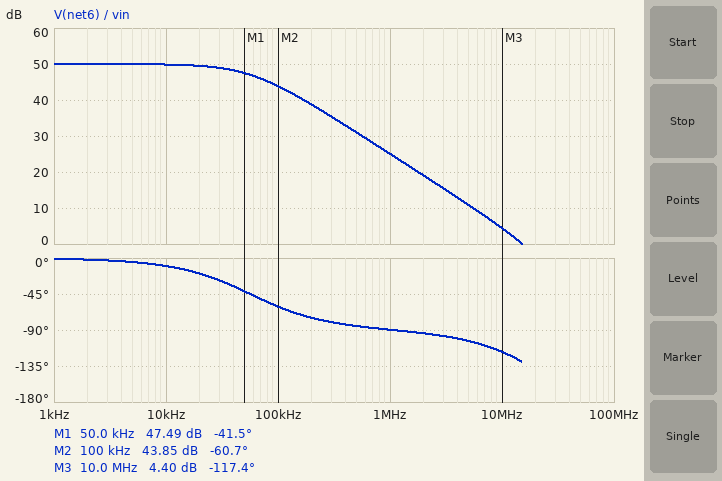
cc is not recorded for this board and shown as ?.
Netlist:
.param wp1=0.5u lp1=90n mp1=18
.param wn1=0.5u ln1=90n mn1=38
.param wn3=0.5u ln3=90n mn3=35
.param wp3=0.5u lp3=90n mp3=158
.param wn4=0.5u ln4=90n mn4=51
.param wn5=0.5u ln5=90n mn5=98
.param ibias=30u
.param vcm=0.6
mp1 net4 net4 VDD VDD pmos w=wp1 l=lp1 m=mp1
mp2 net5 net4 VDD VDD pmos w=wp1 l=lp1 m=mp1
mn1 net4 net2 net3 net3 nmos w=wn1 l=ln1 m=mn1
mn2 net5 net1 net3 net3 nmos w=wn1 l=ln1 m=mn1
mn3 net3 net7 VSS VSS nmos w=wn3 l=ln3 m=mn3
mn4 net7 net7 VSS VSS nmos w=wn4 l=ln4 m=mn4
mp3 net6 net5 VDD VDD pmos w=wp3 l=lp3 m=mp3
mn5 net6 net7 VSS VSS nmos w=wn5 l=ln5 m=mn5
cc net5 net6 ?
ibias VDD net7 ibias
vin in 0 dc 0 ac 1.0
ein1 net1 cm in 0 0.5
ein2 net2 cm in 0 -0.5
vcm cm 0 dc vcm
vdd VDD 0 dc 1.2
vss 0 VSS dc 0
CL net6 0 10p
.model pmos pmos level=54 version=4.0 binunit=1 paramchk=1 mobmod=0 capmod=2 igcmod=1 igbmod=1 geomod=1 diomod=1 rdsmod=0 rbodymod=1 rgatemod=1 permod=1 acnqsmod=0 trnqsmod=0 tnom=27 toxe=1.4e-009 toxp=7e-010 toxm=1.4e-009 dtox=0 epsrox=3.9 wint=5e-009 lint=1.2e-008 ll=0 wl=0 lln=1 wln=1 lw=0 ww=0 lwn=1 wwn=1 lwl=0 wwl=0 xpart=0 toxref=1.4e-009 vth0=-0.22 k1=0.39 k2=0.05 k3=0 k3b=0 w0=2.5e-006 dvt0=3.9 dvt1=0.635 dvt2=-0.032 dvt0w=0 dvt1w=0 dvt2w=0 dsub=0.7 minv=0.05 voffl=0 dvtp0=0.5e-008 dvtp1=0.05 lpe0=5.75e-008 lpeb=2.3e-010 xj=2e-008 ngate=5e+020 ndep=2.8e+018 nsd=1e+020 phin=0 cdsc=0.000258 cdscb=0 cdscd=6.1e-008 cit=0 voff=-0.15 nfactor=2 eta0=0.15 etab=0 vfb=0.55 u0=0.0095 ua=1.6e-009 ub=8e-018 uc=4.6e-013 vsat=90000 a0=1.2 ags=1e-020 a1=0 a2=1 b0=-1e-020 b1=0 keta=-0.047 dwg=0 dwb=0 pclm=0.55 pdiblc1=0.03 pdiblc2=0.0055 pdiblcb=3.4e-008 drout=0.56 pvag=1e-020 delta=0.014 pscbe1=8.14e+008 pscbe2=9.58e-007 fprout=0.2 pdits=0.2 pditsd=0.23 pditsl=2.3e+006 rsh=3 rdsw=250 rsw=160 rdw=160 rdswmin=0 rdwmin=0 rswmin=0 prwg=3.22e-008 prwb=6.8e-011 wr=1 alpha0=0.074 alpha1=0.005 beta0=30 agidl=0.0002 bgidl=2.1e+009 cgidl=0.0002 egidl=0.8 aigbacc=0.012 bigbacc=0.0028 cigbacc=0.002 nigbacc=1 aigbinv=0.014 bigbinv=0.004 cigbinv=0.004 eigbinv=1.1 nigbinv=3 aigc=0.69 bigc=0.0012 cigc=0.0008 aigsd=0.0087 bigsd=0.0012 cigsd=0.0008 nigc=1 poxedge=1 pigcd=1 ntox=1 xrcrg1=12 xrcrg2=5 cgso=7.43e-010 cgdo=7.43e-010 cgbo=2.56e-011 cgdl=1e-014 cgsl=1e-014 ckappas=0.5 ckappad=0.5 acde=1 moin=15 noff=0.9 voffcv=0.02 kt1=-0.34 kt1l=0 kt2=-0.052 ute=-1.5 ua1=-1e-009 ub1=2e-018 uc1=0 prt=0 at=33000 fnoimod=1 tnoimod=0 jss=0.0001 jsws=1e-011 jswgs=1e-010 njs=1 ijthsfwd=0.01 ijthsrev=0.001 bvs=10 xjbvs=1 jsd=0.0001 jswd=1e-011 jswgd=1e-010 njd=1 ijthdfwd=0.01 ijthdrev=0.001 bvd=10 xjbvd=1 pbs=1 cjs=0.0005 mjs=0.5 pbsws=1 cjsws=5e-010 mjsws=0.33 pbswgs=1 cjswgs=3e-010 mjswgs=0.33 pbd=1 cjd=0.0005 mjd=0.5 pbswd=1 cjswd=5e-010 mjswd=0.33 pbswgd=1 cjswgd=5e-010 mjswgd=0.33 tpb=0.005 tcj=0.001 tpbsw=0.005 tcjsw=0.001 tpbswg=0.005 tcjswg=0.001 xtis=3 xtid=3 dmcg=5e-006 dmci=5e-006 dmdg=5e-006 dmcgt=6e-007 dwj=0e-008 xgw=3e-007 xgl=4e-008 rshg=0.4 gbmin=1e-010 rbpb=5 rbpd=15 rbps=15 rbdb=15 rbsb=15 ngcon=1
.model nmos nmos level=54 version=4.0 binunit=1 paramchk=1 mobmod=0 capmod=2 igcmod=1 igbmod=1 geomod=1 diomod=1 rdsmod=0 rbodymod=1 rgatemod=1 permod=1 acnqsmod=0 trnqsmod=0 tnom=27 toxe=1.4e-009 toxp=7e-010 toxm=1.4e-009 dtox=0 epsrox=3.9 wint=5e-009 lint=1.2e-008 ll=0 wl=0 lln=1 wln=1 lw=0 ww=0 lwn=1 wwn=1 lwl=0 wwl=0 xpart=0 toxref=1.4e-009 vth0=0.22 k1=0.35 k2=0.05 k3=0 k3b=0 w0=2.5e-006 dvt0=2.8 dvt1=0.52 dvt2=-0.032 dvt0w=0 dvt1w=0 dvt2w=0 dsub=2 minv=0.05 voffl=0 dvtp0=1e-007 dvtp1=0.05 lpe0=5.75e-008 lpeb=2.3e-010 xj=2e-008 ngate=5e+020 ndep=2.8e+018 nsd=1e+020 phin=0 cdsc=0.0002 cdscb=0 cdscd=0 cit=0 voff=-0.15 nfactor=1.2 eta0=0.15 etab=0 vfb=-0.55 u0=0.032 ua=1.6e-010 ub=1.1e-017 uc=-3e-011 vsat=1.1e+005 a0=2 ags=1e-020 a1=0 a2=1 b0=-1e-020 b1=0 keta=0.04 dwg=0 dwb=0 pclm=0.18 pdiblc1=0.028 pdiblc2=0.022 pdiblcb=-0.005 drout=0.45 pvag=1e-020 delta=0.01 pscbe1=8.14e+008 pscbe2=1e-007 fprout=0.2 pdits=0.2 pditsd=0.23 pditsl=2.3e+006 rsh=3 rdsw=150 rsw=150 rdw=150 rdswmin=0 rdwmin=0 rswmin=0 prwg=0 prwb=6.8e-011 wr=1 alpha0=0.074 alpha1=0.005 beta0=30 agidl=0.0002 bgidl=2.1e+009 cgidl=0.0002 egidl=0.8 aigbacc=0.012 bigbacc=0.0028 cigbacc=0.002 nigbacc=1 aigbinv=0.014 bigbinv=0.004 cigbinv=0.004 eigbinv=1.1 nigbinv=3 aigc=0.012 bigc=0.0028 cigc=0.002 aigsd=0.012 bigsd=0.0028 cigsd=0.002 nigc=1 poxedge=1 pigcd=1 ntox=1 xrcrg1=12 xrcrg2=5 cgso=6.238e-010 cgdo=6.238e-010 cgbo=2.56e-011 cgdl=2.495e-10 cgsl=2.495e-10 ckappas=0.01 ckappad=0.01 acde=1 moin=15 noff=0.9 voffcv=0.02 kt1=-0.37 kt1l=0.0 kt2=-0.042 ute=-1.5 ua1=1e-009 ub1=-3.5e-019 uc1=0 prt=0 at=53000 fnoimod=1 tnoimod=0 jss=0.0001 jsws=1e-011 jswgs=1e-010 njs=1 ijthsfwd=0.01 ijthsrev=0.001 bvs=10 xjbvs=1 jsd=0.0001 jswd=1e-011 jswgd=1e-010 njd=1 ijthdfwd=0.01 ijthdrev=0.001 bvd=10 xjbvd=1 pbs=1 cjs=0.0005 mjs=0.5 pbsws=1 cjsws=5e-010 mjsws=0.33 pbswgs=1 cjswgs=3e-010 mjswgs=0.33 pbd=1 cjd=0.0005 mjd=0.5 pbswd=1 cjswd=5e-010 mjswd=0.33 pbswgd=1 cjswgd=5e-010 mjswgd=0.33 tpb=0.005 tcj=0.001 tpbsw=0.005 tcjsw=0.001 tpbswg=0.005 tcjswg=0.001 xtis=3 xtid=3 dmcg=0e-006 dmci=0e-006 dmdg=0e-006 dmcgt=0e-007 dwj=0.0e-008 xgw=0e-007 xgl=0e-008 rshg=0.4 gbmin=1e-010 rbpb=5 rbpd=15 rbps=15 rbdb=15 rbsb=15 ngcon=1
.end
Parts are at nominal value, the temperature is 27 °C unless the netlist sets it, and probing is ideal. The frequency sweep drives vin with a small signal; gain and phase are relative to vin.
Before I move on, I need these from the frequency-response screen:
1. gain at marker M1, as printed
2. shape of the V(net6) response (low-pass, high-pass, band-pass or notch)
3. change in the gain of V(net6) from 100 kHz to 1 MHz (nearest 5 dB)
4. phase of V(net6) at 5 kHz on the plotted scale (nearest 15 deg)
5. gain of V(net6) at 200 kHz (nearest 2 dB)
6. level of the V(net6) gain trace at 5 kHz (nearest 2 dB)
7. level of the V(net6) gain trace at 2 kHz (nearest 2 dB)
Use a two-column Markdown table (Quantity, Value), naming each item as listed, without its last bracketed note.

| Quantity | Value |
|---|---|
| gain at marker M1, as printed | 47.49 dB |
| shape of the V(net6) response | low-pass |
| change in the gain of V(net6) from 100 kHz to 1 MHz | -20 dB |
| phase of V(net6) at 5 kHz on the plotted scale | 0 deg |
| gain of V(net6) at 200 kHz | 38 dB |
| level of the V(net6) gain trace at 5 kHz | 50 dB |
| level of the V(net6) gain trace at 2 kHz | 50 dB |
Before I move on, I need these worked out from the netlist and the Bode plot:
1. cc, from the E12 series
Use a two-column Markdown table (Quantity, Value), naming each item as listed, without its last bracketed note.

| Quantity | Value |
|---|---|
| cc, from the E12 series | 1.8 pF |
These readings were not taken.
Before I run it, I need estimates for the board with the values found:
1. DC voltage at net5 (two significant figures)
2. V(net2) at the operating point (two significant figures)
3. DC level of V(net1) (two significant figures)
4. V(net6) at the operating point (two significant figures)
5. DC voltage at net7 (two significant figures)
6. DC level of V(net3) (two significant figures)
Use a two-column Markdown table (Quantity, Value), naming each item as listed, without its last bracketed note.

| Quantity | Value |
|---|---|
| DC voltage at net5 | 870 mV |
| V(net2) at the operating point | 600 mV |
| DC level of V(net1) | 600 mV |
| V(net6) at the operating point | 940 mV |
| DC voltage at net7 | 300 mV |
| DC level of V(net3) | 340 mV |
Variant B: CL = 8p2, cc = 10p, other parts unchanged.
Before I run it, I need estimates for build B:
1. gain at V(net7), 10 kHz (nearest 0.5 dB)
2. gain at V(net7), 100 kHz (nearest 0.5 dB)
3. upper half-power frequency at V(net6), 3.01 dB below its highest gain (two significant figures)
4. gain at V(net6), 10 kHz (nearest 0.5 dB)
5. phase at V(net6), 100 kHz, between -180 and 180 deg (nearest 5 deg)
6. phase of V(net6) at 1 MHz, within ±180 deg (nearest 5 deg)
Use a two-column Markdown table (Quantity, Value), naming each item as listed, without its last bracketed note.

| Quantity | Value |
|---|---|
| gain at V(net7), 10 kHz | 10.5 dB |
| gain at V(net7), 100 kHz | -6.5 dB |
| upper half-power frequency at V(net6), 3.01 dB below its highest gain | 11 kHz |
| gain at V(net6), 10 kHz | 47.5 dB |
| phase at V(net6), 100 kHz, between -180 and 180 deg | -85 deg |
| phase of V(net6) at 1 MHz, within ±180 deg | -95 deg |
